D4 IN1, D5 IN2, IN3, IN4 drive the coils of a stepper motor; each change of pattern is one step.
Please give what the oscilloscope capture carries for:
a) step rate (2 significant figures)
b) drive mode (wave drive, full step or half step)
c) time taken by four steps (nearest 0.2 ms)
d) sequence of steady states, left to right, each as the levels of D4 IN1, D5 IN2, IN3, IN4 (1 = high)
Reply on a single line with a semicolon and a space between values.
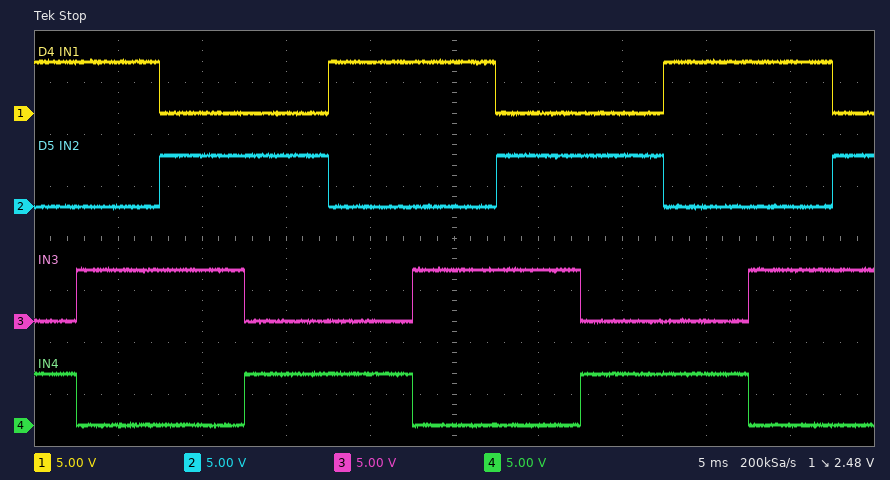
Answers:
200 steps/s; full step; 20.0 ms; 1001 1010 0110 0101 1001 1010 0110 0101 1001 1010 0110
